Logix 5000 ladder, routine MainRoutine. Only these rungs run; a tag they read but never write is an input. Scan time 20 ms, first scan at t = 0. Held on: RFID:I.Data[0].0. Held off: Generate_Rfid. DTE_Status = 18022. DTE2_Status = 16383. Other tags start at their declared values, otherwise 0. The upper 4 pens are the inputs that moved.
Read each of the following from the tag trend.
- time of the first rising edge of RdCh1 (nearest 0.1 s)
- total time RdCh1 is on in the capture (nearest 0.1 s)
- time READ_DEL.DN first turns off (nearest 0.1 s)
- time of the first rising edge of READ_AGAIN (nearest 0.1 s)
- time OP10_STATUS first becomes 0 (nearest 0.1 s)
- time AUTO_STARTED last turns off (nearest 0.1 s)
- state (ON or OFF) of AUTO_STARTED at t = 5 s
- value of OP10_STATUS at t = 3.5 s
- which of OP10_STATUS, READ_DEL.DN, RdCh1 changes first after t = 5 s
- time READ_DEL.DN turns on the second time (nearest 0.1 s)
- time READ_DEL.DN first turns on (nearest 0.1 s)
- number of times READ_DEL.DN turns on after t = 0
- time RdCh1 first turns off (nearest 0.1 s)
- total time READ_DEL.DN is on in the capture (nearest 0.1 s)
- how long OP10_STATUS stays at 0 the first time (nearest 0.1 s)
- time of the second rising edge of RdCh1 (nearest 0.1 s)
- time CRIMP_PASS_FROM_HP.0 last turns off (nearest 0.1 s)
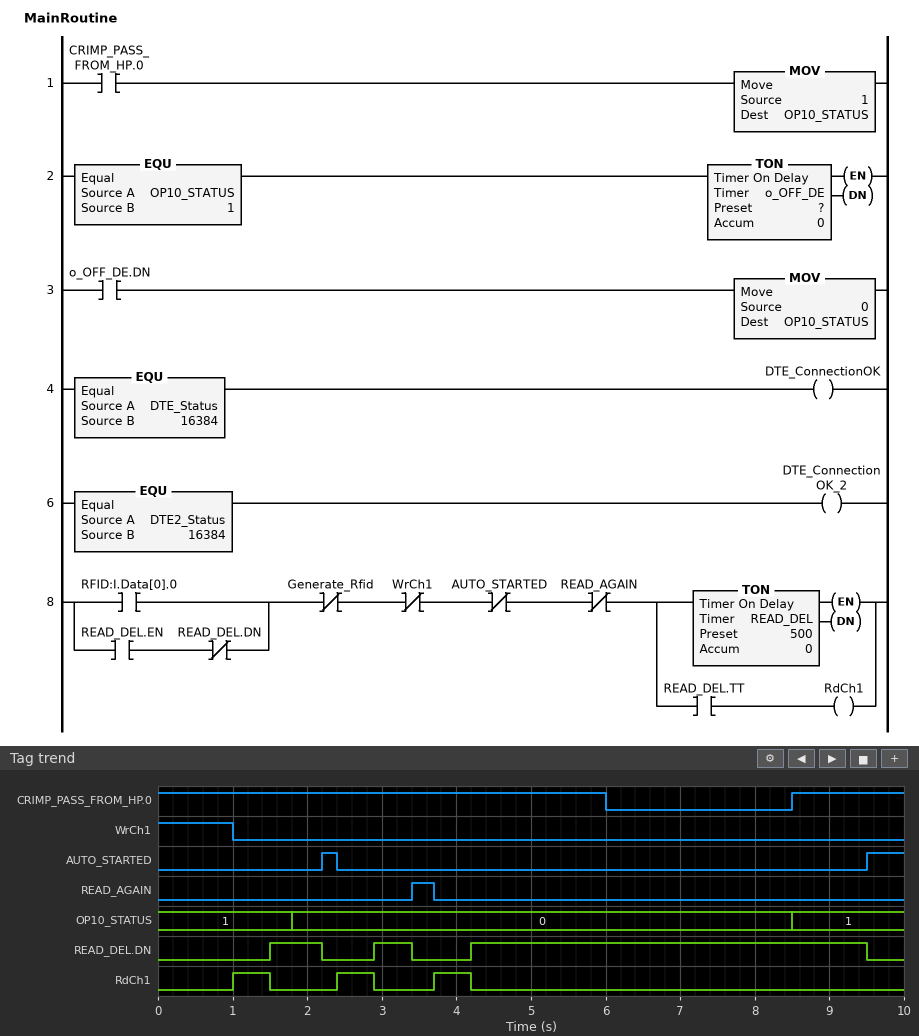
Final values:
1.0 s
1.5 s
2.2 s
3.4 s
1.8 s
2.4 s
OFF
0
OP10_STATUS
2.9 s
1.5 s
3
1.5 s
6.5 s
6.7 s
2.4 s
6.0 s
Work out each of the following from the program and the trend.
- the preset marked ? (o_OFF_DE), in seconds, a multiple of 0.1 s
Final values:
1.8 s
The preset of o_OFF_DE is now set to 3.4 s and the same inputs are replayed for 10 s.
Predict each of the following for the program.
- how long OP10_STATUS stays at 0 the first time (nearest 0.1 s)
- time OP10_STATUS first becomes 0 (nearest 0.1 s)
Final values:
5.1 s
3.4 s
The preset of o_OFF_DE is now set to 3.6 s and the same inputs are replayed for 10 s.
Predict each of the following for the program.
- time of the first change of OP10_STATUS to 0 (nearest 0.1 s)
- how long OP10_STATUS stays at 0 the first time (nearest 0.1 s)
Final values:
3.6 s
4.9 s
